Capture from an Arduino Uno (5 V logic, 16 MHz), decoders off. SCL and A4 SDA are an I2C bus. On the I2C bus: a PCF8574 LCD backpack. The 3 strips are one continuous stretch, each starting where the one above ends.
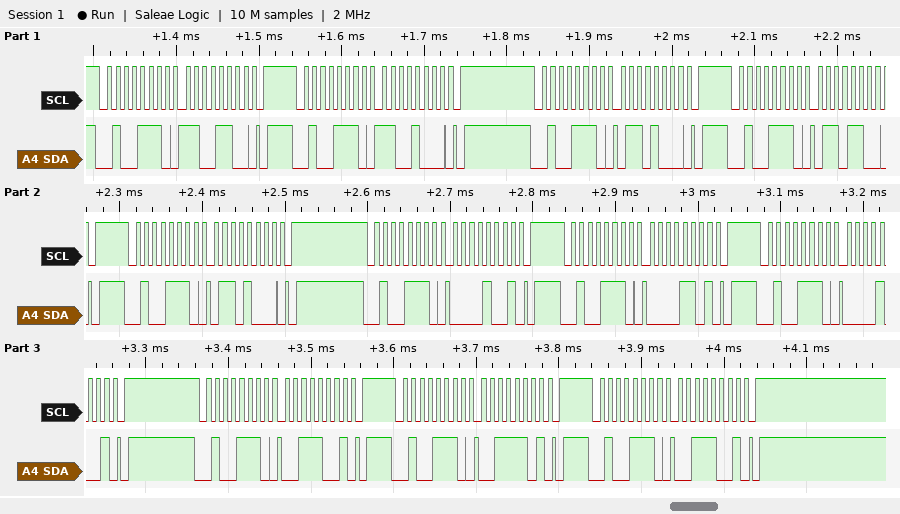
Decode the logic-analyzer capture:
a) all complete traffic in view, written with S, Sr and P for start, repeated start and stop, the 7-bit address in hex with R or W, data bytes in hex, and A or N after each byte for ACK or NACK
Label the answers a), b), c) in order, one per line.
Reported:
a) S 27W A CC A P S 27W A C8 A P S 27W A 68 A P S 27W A 6C A P S 27W A 68 A P S 27W A 09 A P S 27W A 0D A P S 27W A 09 A P S 27W A 39 A P S 27W A 3D A P S 27W A 39 A P
